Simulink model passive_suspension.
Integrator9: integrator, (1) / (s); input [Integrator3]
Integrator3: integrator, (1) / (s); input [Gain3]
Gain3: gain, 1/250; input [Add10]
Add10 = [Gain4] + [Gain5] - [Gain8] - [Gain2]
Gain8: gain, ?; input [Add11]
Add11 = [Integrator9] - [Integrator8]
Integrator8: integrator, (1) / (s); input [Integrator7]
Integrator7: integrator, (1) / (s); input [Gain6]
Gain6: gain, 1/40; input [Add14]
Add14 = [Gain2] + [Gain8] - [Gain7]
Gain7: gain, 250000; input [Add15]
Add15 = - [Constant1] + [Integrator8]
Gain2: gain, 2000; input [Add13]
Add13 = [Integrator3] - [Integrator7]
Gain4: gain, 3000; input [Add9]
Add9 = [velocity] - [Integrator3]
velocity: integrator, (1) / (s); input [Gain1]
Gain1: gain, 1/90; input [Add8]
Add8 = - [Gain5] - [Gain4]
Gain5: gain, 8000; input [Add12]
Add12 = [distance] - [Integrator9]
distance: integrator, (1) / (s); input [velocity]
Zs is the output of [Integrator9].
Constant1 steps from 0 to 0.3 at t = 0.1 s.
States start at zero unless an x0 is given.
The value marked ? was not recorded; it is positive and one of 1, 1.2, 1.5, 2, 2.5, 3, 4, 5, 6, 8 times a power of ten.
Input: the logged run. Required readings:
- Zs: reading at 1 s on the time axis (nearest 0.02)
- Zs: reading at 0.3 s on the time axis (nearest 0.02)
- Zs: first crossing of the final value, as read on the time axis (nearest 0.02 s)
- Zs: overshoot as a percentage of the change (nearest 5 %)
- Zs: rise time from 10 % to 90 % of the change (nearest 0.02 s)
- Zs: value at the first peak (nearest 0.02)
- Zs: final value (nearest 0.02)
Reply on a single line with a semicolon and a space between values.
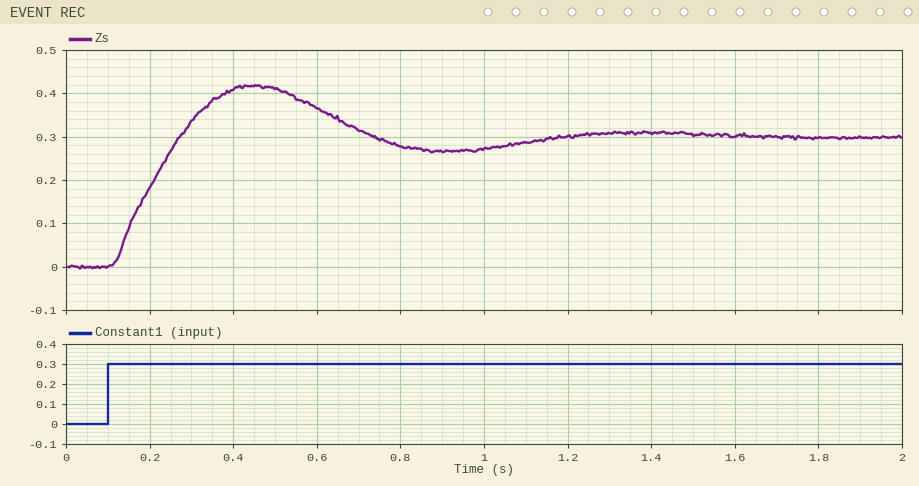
0.28; 0.34; 0.28 s; 40 %; 0.12 s; 0.42; 0.30
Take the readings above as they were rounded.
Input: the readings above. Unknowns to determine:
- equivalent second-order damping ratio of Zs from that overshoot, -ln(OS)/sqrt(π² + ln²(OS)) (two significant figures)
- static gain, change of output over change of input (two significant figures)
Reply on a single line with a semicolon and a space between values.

0.28; 1.0
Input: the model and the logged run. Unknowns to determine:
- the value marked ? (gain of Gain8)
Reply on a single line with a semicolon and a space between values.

20000
